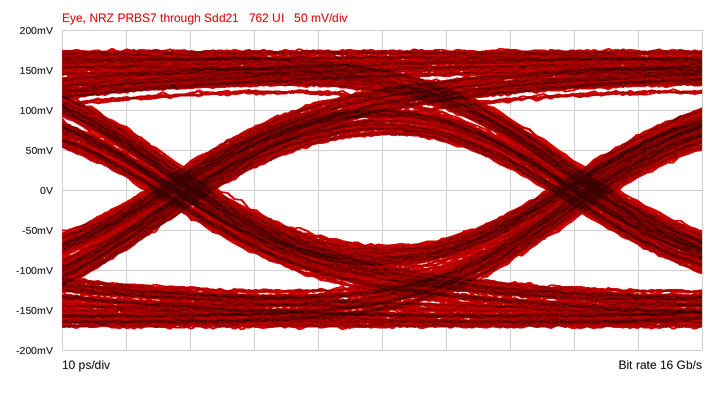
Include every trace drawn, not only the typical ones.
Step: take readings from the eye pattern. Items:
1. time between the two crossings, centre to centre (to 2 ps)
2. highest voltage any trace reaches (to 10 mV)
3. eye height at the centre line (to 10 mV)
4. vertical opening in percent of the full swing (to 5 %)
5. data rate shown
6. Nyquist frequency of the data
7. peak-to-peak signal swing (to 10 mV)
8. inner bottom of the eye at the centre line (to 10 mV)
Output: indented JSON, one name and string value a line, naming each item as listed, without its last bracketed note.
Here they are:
{
  "time between the two crossings, centre to centre": "62 ps",
  "highest voltage any trace reaches": "180 mV",
  "eye height at the centre line": "140 mV",
  "vertical opening in percent of the full swing": "40 %",
  "data rate shown": "16 Gb/s",
  "Nyquist frequency of the data": "8 GHz",
  "peak-to-peak signal swing": "350 mV",
  "inner bottom of the eye at the centre line": "-70 mV"
}
